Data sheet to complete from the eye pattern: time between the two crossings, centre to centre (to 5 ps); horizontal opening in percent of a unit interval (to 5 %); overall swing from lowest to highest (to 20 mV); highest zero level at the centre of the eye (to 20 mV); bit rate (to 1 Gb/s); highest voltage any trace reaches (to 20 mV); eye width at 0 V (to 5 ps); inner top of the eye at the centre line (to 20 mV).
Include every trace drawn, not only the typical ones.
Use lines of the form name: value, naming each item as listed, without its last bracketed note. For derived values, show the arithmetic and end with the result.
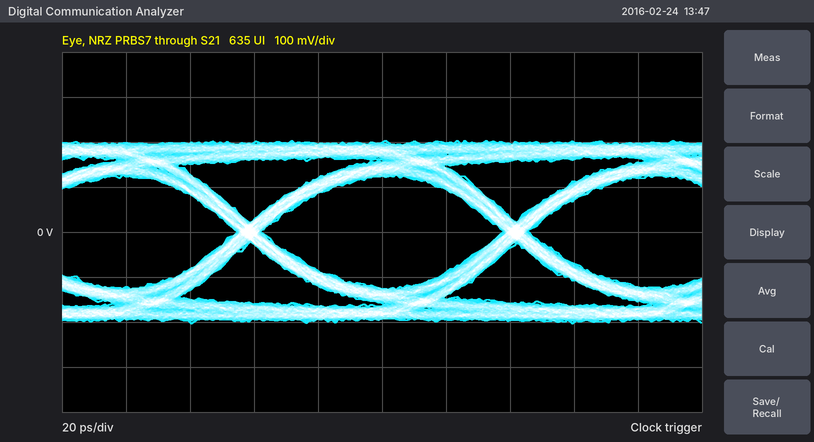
time between the two crossings, centre to centre: 85 ps
horizontal opening in percent of a unit interval: 75 ps / 85 ps ≈ 88.2 %, so 90 % to the nearest 5 %
overall swing from lowest to highest: 400 mV
highest zero level at the centre of the eye: -120 mV
bit rate: 12 Gb/s
highest voltage any trace reaches: 200 mV
eye width at 0 V: 75 ps
inner top of the eye at the centre line: 120 mV
